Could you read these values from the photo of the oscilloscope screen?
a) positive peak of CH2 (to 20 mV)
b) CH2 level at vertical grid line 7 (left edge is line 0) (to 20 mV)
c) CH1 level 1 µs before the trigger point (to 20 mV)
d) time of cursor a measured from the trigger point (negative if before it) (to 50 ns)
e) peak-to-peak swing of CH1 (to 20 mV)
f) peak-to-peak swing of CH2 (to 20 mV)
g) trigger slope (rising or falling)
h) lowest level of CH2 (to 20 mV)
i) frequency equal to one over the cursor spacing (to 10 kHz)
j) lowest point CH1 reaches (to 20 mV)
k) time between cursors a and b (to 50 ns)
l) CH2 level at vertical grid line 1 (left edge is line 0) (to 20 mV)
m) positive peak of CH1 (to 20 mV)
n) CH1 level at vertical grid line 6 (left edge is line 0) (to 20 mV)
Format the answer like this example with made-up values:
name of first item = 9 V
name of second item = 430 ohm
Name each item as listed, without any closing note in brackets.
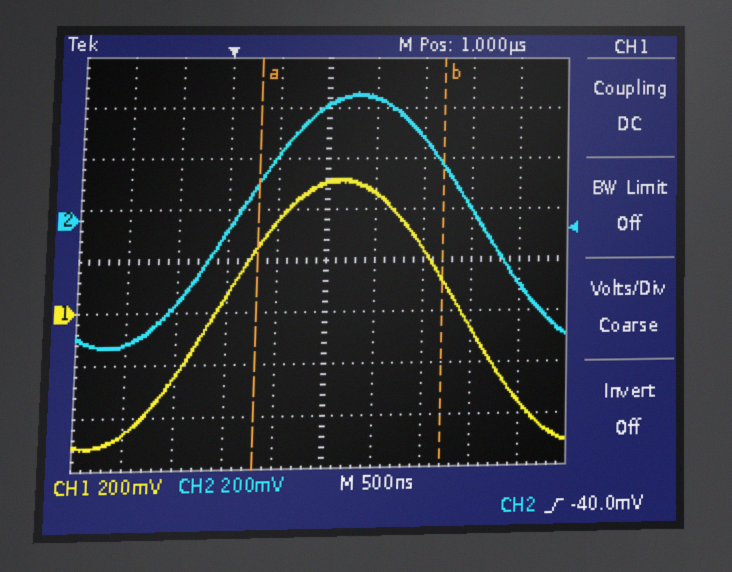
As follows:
positive peak of CH2 = 500 mV
CH2 level at vertical grid line 7 (left edge is line 0) = 320 mV
CH1 level 1 µs before the trigger point = -460 mV
time of cursor a measured from the trigger point (negative if before it) = +300 ns
peak-to-peak swing of CH1 = 1.04 V
peak-to-peak swing of CH2 = 1.00 V
trigger slope = rising
lowest level of CH2 = -500 mV
frequency equal to one over the cursor spacing = 530 kHz
lowest point CH1 reaches = -520 mV
time between cursors a and b = 1.90 µs
CH2 level at vertical grid line 1 (left edge is line 0) = -480 mV
positive peak of CH1 = 520 mV
CH1 level at vertical grid line 6 (left edge is line 0) = 460 mV
